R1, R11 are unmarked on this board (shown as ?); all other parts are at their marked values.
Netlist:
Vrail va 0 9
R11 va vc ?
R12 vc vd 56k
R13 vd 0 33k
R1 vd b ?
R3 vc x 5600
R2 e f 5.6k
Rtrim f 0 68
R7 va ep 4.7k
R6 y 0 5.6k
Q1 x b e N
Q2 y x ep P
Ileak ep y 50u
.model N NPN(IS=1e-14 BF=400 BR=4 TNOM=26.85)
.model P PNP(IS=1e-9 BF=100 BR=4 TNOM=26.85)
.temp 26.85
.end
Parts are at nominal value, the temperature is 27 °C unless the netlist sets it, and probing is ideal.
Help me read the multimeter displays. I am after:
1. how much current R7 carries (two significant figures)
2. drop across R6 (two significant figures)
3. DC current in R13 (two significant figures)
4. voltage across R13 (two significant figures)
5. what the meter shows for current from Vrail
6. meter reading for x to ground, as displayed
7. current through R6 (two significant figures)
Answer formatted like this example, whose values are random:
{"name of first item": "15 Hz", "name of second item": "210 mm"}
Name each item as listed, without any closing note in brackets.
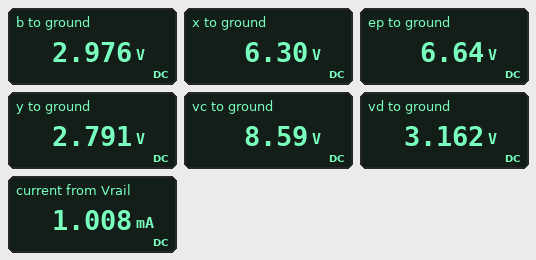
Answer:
{"how much current R7 carries": "500 µA", "drop across R6": "2.8 V", "DC current in R13": "96 µA", "voltage across R13": "3.2 V", "what the meter shows for current from Vrail": "1.008 mA", "meter reading for x to ground, as displayed": "6.30 V", "current through R6": "500 µA"}
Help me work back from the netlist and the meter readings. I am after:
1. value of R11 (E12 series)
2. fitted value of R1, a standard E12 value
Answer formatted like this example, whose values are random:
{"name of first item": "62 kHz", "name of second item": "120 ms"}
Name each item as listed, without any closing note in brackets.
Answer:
{"value of R11": "820 Ω", "fitted value of R1, a standard E12 value": "180 kΩ"}
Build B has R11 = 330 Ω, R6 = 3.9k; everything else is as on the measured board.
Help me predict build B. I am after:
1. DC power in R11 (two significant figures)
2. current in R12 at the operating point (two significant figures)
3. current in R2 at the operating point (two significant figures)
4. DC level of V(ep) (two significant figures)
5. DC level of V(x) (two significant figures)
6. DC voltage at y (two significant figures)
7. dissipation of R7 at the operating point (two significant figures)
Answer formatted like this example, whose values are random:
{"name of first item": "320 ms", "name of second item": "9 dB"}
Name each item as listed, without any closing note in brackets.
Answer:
{"DC power in R11": "90 µW", "current in R12 at the operating point": "100 µA", "current in R2 at the operating point": "430 µA", "DC level of V(ep)": "6.8 V", "DC level of V(x)": "6.5 V", "DC voltage at y": "1.8 V", "dissipation of R7 at the operating point": "1.0 mW"}
